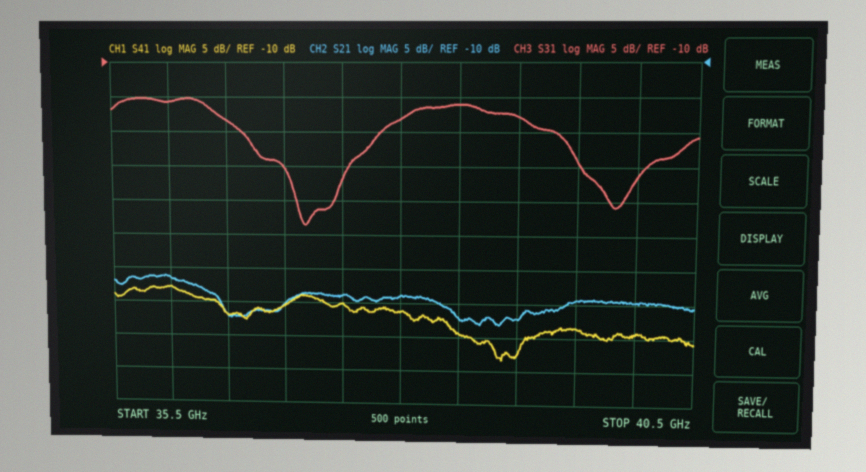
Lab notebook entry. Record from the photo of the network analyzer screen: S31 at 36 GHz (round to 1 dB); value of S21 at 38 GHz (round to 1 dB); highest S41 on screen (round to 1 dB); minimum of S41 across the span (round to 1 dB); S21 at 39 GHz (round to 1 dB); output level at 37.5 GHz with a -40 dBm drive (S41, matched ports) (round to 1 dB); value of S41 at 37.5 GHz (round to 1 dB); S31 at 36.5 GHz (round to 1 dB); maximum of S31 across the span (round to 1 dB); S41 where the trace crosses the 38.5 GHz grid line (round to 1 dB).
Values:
-16 dB
-44 dB
-43 dB
-53 dB
-47 dB
-85 dBm
-45 dB
-18 dB
-15 dB
-49 dB
